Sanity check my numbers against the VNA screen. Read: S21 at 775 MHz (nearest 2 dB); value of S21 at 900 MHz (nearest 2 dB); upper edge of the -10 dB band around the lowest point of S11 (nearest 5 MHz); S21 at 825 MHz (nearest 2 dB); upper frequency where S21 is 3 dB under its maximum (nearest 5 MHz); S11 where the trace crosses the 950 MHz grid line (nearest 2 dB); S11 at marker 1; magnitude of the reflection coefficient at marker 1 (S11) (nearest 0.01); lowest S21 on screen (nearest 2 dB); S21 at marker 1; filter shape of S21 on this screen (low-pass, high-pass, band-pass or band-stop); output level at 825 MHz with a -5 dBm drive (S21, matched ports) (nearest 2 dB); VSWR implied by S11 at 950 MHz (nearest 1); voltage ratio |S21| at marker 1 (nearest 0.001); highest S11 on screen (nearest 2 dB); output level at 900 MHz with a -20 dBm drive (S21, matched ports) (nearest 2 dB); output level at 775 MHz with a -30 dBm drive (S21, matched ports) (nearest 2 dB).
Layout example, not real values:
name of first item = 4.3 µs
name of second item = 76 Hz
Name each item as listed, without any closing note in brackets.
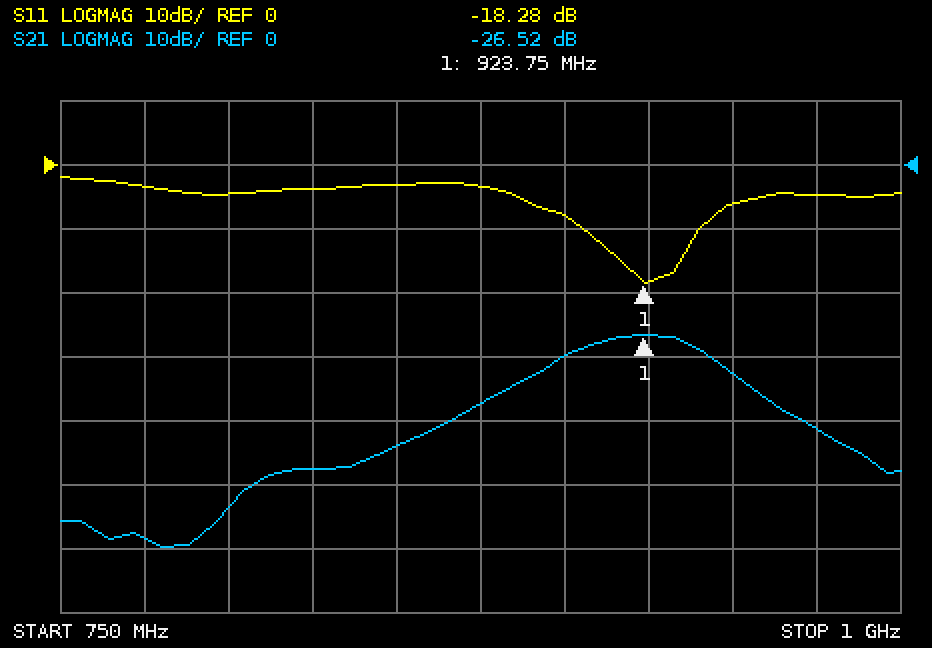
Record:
S21 at 775 MHz = -58 dB
value of S21 at 900 MHz = -30 dB
upper edge of the -10 dB band around the lowest point of S11 = 940 MHz
S21 at 825 MHz = -48 dB
upper frequency where S21 is 3 dB under its maximum = 940 MHz
S11 where the trace crosses the 950 MHz grid line = -6 dB
S11 at marker 1 = -18.28 dB
magnitude of the reflection coefficient at marker 1 (S11) = 0.12
lowest S21 on screen = -60 dB
S21 at marker 1 = -26.52 dB
filter shape of S21 on this screen = band-pass
output level at 825 MHz with a -5 dBm drive (S21, matched ports) = -52 dBm
VSWR implied by S11 at 950 MHz = 3
voltage ratio |S21| at marker 1 = 0.047
highest S11 on screen = -2 dB
output level at 900 MHz with a -20 dBm drive (S21, matched ports) = -50 dBm
output level at 775 MHz with a -30 dBm drive (S21, matched ports) = -88 dBm
